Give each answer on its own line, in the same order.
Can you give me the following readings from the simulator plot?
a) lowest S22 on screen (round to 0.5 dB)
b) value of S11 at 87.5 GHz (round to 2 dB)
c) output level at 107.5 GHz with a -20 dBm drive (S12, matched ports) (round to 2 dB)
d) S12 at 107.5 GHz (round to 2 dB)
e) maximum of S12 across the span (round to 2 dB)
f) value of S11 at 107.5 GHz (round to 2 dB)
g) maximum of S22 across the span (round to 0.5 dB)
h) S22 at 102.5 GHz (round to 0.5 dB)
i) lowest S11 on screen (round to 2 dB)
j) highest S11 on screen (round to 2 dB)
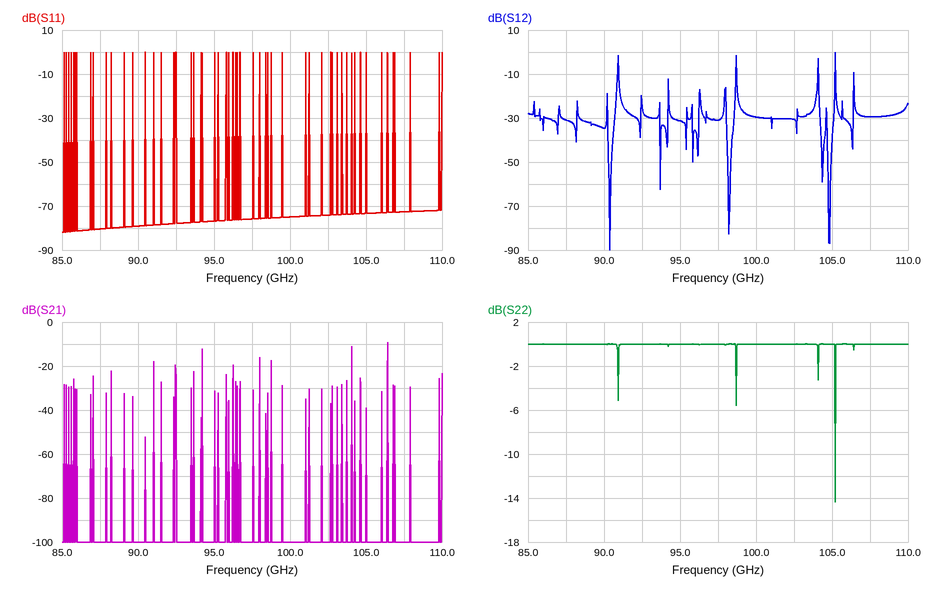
-14.5 dB
-80 dB
-50 dBm
-30 dB
0 dB
-72 dB
0.0 dB
0.0 dB
-82 dB
0 dB
